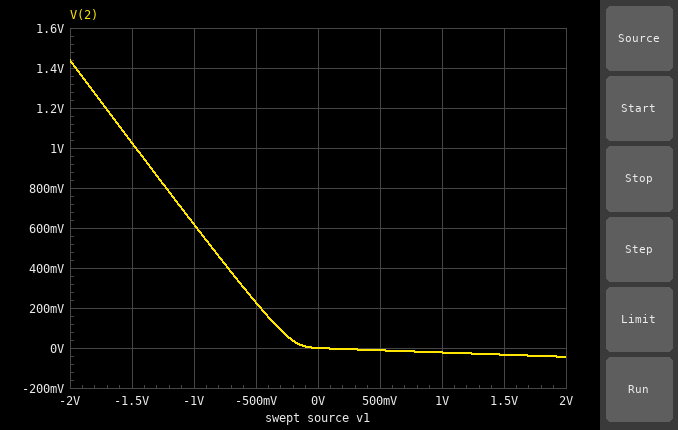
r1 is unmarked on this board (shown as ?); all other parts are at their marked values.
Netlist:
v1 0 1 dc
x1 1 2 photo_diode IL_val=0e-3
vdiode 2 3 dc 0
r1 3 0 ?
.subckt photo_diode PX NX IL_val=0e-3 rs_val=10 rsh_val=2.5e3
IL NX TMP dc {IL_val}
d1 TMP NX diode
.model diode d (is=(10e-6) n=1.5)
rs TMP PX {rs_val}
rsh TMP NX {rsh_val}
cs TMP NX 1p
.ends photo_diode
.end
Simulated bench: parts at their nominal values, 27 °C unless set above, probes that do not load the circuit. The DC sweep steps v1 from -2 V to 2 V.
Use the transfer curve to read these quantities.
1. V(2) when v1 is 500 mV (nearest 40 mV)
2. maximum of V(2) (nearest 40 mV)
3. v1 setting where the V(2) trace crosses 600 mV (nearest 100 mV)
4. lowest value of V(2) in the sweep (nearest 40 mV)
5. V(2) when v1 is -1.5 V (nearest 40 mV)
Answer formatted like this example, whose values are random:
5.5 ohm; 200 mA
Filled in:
0 V; 1.44 V; -1.0 V; -40 mV; 1.04 V
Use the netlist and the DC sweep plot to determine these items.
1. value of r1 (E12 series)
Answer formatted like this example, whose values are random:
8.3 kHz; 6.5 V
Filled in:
56 Ω
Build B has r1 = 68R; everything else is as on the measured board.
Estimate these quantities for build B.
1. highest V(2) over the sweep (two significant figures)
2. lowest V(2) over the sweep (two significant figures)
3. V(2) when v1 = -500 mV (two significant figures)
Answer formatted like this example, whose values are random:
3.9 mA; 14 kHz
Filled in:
1.5 V; -53 mV; 240 mV
